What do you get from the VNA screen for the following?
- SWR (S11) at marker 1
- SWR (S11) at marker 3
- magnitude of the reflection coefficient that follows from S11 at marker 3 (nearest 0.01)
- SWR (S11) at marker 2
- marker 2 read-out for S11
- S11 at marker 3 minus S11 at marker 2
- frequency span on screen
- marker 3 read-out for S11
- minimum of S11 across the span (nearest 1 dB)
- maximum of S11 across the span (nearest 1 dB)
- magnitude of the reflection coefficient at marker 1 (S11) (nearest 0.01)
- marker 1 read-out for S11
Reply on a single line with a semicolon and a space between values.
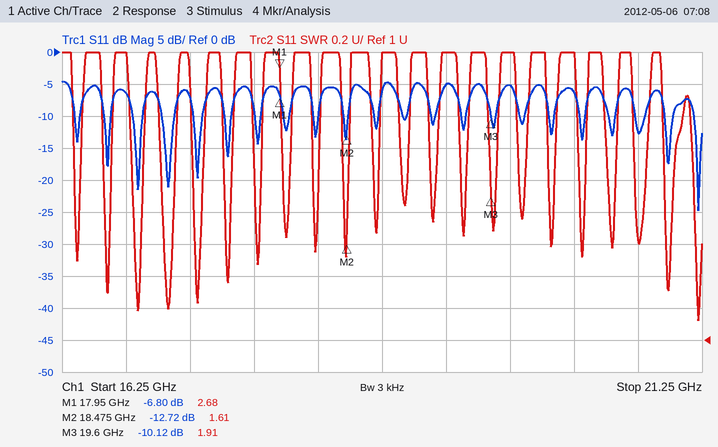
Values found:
2.68; 1.91; 0.31; 1.61; -12.72 dB; 2.60 dB; 5 GHz; -10.12 dB; -25 dB; -5 dB; 0.46; -6.80 dB
